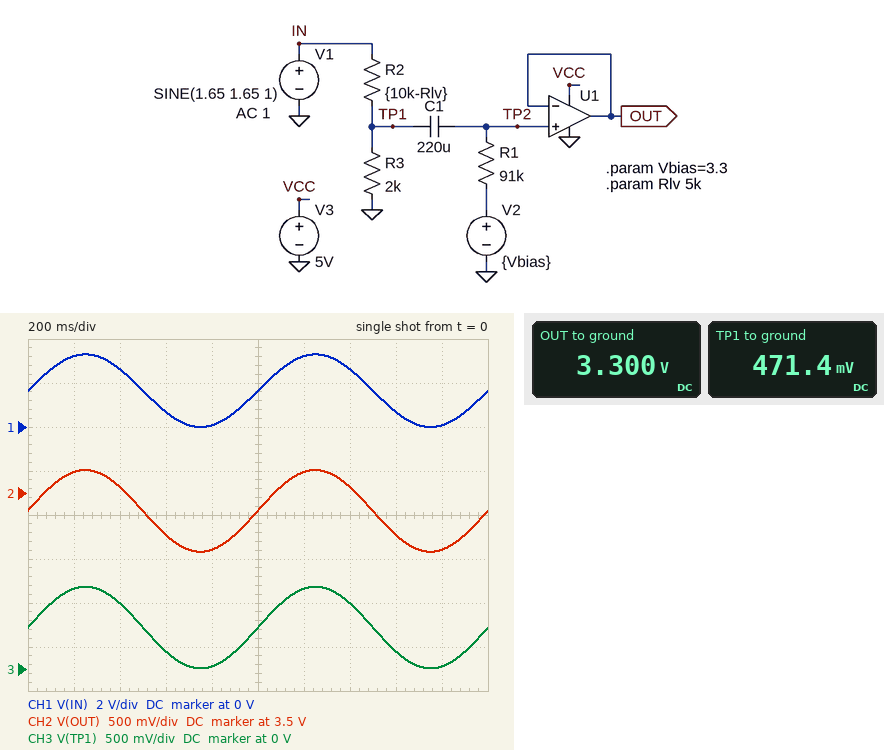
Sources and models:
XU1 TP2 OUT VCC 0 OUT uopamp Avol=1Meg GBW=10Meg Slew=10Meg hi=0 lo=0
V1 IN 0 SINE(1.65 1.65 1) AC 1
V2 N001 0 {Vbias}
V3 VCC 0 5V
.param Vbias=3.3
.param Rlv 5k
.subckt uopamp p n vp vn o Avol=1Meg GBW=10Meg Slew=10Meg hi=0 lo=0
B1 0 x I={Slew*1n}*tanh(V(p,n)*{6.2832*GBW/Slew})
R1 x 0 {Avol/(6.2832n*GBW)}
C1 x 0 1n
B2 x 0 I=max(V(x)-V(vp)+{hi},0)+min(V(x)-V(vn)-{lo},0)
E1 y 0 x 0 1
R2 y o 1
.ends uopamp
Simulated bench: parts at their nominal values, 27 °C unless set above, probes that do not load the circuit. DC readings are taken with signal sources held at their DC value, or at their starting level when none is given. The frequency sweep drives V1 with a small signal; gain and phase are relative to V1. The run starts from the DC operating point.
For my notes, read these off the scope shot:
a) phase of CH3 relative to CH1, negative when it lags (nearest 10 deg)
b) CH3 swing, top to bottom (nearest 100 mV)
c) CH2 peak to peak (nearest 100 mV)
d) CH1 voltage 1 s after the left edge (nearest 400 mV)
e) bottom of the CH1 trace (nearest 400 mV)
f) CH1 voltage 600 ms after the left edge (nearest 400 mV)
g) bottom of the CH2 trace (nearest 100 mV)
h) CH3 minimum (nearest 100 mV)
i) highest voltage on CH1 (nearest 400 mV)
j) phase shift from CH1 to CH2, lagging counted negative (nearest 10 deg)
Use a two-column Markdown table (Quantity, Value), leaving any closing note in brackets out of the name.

| Quantity | Value |
|---|---|
| phase of CH3 relative to CH1, negative when it lags | 0 deg |
| CH3 swing, top to bottom | 900 mV |
| CH2 peak to peak | 900 mV |
| CH1 voltage 1 s after the left edge | 1.6 V |
| bottom of the CH1 trace | 0 V |
| CH1 voltage 600 ms after the left edge | 800 mV |
| bottom of the CH2 trace | 2.8 V |
| CH3 minimum | 0 V |
| highest voltage on CH1 | 3.2 V |
| phase shift from CH1 to CH2, lagging counted negative | 0 deg |
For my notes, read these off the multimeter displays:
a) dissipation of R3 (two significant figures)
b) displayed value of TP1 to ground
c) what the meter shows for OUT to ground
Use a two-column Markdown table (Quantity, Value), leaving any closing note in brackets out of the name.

| Quantity | Value |
|---|---|
| dissipation of R3 | 110 µW |
| displayed value of TP1 to ground | 471.4 mV |
| what the meter shows for OUT to ground | 3.300 V |
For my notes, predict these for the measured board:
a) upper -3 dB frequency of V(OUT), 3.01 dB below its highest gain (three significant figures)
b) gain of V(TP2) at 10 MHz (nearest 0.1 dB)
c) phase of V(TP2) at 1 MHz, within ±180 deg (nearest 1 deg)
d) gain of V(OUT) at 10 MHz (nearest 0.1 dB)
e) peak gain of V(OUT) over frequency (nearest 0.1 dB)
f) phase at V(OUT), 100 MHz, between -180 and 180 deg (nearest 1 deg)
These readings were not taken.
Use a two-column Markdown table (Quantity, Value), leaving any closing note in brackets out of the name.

| Quantity | Value |
|---|---|
| upper -3 dB frequency of V(OUT), 3.01 dB below its highest gain | 10.0 MHz |
| gain of V(TP2) at 10 MHz | -11.0 dB |
| phase of V(TP2) at 1 MHz, within ±180 deg | 0 deg |
| gain of V(OUT) at 10 MHz | -14.0 dB |
| peak gain of V(OUT) over frequency | -11.0 dB |
| phase at V(OUT), 100 MHz, between -180 and 180 deg | -84 deg |
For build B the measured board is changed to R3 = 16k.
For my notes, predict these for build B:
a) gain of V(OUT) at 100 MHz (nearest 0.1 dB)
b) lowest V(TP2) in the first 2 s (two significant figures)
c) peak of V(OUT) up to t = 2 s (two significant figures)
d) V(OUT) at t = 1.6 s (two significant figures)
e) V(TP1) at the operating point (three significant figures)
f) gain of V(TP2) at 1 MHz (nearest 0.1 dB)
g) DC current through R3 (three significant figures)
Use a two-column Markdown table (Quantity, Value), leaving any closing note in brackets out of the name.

| Quantity | Value |
|---|---|
| gain of V(OUT) at 100 MHz | -22.8 dB |
| lowest V(TP2) in the first 2 s | 2.1 V |
| peak of V(OUT) up to t = 2 s | 4.5 V |
| V(OUT) at t = 1.6 s | 2.6 V |
| V(TP1) at the operating point | 1.26 V |
| gain of V(TP2) at 1 MHz | -2.7 dB |
| DC current through R3 | 78.6 µA |
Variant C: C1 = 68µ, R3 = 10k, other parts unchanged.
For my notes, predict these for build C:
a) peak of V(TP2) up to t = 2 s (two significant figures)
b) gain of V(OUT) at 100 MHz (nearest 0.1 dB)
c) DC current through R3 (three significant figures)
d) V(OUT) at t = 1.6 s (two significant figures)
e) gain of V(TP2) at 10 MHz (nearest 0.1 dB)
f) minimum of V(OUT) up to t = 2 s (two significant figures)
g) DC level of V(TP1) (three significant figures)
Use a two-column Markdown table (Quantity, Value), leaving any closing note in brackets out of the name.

| Quantity | Value |
|---|---|
| peak of V(TP2) up to t = 2 s | 4.3 V |
| gain of V(OUT) at 100 MHz | -23.9 dB |
| DC current through R3 | 110 µA |
| V(OUT) at t = 1.6 s | 2.6 V |
| gain of V(TP2) at 10 MHz | -3.8 dB |
| minimum of V(OUT) up to t = 2 s | 2.2 V |
| DC level of V(TP1) | 1.10 V |
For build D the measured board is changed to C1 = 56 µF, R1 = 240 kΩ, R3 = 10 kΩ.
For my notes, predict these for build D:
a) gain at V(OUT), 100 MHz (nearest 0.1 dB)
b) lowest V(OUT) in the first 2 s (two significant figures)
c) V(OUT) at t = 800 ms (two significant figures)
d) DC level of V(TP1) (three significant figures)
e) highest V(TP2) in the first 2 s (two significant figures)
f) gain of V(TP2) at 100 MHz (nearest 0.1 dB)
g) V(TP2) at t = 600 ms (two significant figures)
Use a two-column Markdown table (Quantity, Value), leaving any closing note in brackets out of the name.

| Quantity | Value |
|---|---|
| gain at V(OUT), 100 MHz | -23.7 dB |
| lowest V(OUT) in the first 2 s | 2.2 V |
| V(OUT) at t = 800 ms | 2.3 V |
| DC level of V(TP1) | 1.10 V |
| highest V(TP2) in the first 2 s | 4.4 V |
| gain of V(TP2) at 100 MHz | -3.6 dB |
| V(TP2) at t = 600 ms | 2.6 V |
